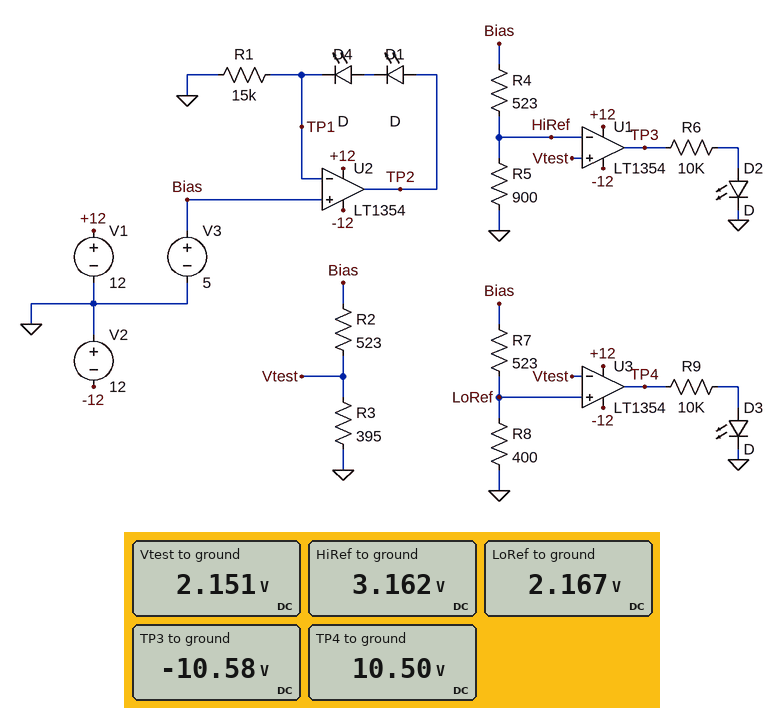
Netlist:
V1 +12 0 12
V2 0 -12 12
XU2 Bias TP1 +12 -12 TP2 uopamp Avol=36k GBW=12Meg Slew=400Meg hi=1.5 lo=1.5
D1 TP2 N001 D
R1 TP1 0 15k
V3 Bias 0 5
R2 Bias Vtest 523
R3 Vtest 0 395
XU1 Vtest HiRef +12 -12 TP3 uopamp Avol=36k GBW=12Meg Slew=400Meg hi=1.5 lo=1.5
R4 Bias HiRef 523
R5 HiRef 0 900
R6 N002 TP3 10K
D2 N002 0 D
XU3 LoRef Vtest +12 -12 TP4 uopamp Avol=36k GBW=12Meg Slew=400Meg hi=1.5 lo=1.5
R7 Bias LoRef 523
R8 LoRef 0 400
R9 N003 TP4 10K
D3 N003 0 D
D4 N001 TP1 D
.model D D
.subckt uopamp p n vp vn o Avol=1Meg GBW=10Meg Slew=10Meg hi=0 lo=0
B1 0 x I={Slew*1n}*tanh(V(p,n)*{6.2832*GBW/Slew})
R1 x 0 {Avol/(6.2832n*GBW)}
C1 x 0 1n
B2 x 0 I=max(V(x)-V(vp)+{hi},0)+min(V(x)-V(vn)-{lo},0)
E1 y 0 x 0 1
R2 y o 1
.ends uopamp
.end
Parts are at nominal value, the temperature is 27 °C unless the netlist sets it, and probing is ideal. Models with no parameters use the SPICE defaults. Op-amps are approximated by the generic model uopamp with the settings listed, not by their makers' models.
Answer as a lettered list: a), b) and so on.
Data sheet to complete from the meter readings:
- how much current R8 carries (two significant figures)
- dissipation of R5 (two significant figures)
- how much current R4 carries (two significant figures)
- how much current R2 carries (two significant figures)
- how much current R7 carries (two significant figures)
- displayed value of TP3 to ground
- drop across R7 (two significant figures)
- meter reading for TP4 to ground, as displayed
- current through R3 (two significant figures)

a) 5.4 mA
b) 11 mW
c) 3.5 mA
d) 5.4 mA
e) 5.4 mA
f) -10.58 V
g) 2.8 V
h) 10.50 V
i) 5.4 mA
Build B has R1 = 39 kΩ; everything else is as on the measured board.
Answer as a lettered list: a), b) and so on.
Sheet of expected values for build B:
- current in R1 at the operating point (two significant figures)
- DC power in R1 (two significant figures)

a) 130 µA
b) 640 µW
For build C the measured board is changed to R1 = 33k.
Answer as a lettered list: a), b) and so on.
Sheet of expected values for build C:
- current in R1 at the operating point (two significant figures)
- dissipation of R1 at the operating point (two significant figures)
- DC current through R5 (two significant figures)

a) 150 µA
b) 760 µW
c) 3.5 mA
